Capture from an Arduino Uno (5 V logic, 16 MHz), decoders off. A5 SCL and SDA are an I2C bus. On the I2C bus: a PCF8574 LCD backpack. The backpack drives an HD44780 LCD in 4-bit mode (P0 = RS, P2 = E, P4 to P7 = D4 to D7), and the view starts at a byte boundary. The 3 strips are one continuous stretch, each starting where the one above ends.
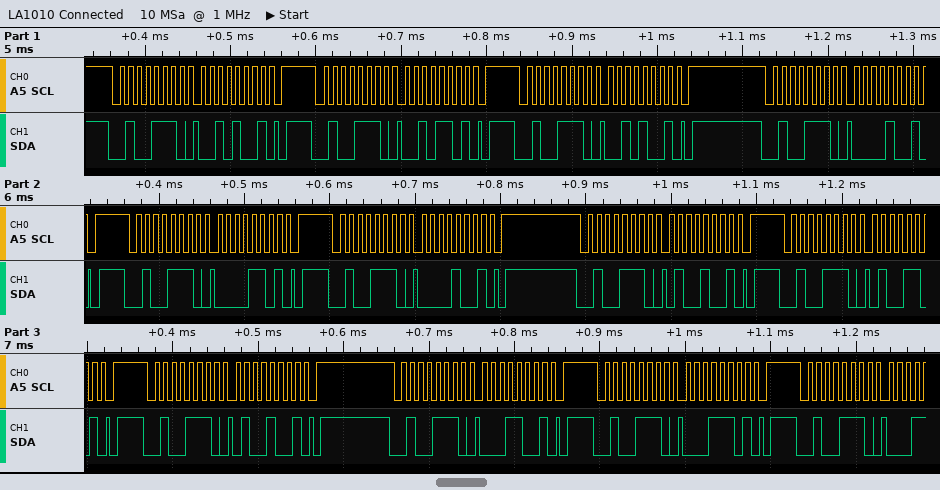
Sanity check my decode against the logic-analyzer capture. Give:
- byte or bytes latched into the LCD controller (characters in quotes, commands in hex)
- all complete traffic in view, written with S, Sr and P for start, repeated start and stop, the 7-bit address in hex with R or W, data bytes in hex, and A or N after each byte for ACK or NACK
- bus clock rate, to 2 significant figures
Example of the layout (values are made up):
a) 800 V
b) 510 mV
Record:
a) ' '
b) S 27W A 29 A P S 27W A 2D A P S 27W A 29 A P S 27W A 09 A P S 27W A 0D A P S 27W A 09 A P S 27W A 49 A P S 27W A 4D A P S 27W A 49 A P S 27W A 19 A P S 27W A 1D A P S 27W A
c) 100 kHz
